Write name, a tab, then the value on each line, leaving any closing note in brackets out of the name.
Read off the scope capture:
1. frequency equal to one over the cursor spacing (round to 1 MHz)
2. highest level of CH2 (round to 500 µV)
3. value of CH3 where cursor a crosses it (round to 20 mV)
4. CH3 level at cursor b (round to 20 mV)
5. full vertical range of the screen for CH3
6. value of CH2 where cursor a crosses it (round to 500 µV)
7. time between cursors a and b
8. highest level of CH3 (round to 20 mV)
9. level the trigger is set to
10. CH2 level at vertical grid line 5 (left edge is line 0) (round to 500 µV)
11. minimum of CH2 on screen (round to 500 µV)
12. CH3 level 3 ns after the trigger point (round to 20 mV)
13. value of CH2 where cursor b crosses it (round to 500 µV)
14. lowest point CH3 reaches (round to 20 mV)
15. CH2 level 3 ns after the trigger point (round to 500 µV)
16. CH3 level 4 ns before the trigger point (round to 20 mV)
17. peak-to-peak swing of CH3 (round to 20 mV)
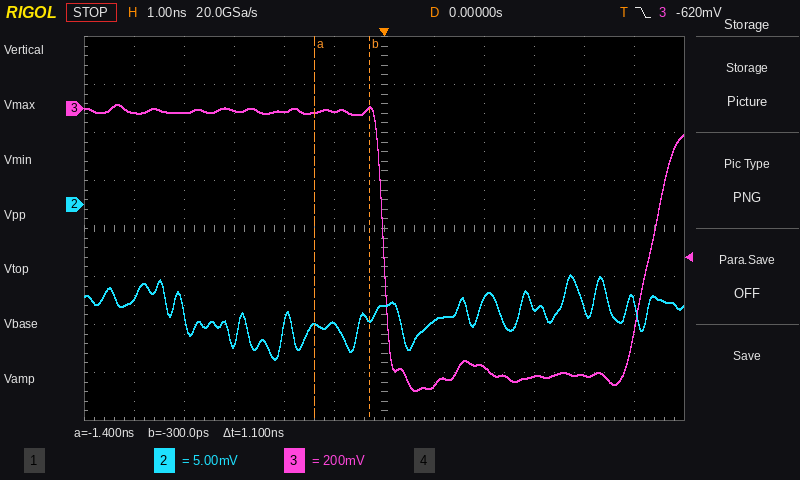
frequency equal to one over the cursor spacing	909 MHz
highest level of CH2	-7.5 mV
value of CH3 where cursor a crosses it	-20 mV
CH3 level at cursor b	0 mV
full vertical range of the screen for CH3	1.6 V
value of CH2 where cursor a crosses it	-12.5 mV
time between cursors a and b	1.1 ns
highest level of CH3	20 mV
level the trigger is set to	-620 mV
CH2 level at vertical grid line 5 (left edge is line 0)	-12.5 mV
minimum of CH2 on screen	-16.0 mV
CH3 level 3 ns after the trigger point	-1.12 V
value of CH2 where cursor b crosses it	-12.0 mV
lowest point CH3 reaches	-1.18 V
CH2 level 3 ns after the trigger point	-10.5 mV
CH3 level 4 ns before the trigger point	-20 mV
peak-to-peak swing of CH3	1.20 V
